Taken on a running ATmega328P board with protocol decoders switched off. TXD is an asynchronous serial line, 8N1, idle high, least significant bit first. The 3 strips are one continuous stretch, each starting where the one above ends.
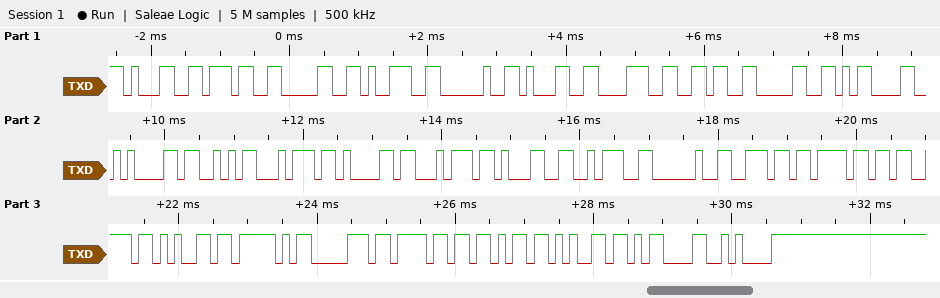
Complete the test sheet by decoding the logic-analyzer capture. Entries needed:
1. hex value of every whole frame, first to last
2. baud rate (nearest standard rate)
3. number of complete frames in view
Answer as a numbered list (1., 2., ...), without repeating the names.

1. 31 37 30 39 20 31 38 36 30 0D 0A 53 74 61 74 31 3A 20 6E 6F 73 65 5F 70 6F 6B 65 0D 0A
2. 9600 baud
3. 29
